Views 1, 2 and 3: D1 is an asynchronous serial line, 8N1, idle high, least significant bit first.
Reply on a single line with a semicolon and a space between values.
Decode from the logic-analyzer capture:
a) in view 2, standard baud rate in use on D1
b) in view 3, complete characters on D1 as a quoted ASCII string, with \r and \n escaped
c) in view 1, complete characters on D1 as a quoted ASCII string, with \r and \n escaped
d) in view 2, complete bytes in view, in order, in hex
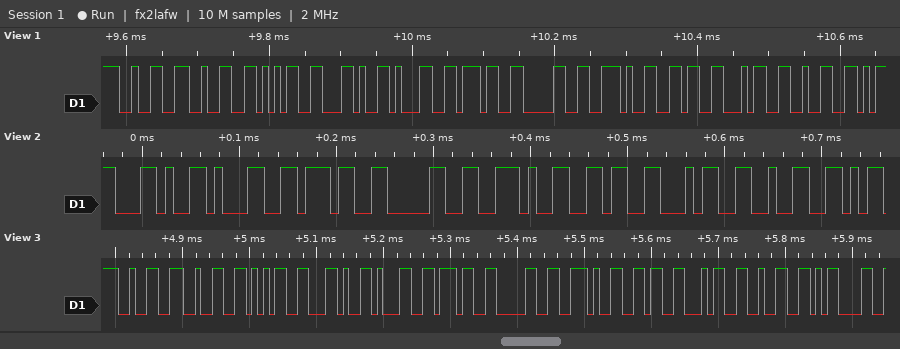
115200 baud; "225,170.642\r"; "225,170.642"; 0x2C 0x31 0x37 0x30 0x2E 0x36 0x34 0x32
